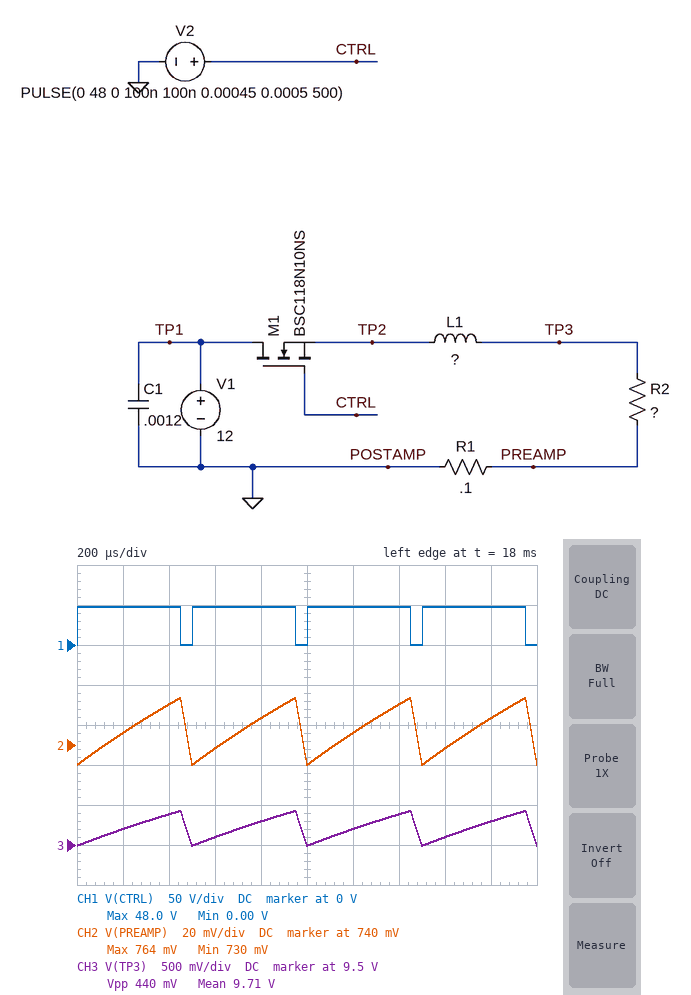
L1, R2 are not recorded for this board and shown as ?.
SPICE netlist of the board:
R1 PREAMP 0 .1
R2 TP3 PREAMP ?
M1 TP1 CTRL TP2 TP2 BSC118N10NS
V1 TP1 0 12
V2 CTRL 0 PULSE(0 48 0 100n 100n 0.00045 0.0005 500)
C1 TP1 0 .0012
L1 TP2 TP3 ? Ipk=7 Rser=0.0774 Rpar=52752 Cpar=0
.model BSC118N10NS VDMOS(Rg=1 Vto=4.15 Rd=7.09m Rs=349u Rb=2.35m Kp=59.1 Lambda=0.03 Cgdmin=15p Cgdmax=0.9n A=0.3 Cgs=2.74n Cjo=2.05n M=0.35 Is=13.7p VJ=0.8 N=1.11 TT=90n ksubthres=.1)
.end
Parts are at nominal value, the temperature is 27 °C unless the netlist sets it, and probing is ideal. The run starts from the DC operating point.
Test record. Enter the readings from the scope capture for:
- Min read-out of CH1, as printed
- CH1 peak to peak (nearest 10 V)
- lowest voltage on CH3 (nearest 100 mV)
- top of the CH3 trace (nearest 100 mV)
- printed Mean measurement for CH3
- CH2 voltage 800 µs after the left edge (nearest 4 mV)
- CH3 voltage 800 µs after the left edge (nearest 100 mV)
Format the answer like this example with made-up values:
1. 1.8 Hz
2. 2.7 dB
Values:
1. 0.00 V
2. 50 V
3. 9.5 V
4. 9.9 V
5. 9.71 V
6. 752 mV
7. 9.8 V
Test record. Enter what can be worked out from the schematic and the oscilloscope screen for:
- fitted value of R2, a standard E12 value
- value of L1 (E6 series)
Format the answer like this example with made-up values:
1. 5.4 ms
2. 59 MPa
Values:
1. 1.2 Ω
2. 2.2 mH
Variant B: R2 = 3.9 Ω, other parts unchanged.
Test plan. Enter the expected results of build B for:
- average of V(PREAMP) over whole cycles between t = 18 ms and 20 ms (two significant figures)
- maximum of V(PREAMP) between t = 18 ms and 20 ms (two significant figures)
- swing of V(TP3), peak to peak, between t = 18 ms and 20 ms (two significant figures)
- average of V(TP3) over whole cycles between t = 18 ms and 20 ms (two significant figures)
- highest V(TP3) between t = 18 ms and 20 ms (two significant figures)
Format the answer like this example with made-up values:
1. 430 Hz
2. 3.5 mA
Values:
1. 250 mV
2. 270 mV
3. 1.3 V
4. 10 V
5. 11 V
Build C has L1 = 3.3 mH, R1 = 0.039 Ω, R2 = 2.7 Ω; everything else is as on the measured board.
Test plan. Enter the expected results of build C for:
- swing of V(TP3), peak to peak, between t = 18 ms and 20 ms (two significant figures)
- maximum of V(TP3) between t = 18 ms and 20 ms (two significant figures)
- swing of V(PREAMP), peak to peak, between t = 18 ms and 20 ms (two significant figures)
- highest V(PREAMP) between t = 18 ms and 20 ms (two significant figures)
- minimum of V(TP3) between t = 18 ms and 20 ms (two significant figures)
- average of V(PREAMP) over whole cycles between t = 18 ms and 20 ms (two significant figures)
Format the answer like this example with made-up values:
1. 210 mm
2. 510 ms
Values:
1. 610 mV
2. 10 V
3. 8.7 mV
4. 150 mV
5. 9.7 V
6. 140 mV
